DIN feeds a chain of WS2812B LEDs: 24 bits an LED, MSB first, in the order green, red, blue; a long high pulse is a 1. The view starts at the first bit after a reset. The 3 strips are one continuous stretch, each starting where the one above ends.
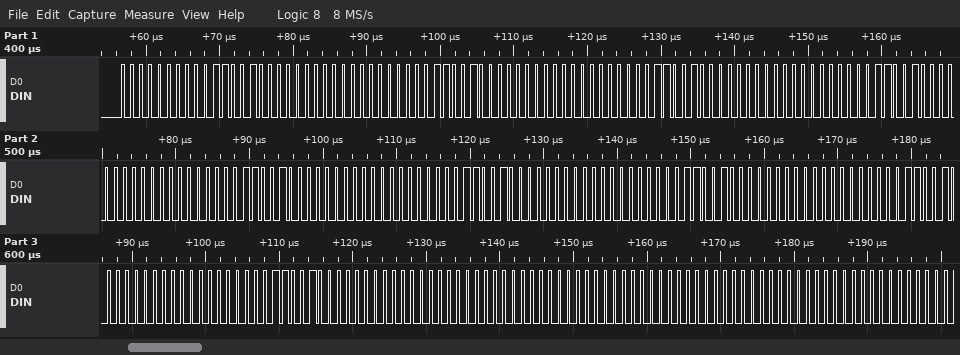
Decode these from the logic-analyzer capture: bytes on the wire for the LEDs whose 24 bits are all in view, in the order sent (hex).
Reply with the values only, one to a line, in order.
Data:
00 32 00 00 32 00 00 32 00 00 32 00 00 32 00 00 32 00 00 32 00 00 32 00 00 32 00 00 00 00 00 00 00
